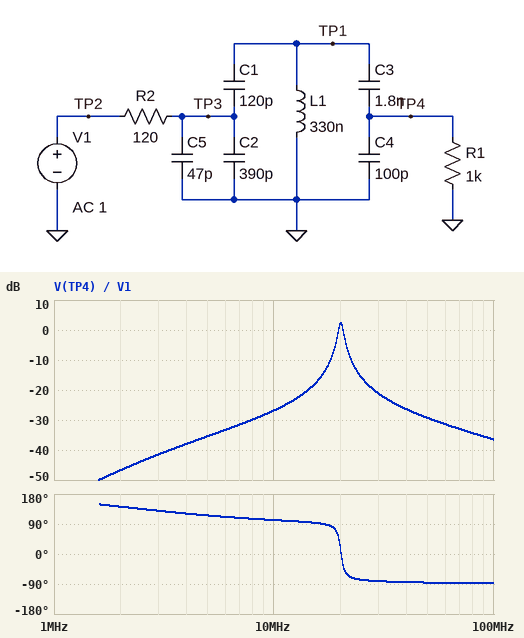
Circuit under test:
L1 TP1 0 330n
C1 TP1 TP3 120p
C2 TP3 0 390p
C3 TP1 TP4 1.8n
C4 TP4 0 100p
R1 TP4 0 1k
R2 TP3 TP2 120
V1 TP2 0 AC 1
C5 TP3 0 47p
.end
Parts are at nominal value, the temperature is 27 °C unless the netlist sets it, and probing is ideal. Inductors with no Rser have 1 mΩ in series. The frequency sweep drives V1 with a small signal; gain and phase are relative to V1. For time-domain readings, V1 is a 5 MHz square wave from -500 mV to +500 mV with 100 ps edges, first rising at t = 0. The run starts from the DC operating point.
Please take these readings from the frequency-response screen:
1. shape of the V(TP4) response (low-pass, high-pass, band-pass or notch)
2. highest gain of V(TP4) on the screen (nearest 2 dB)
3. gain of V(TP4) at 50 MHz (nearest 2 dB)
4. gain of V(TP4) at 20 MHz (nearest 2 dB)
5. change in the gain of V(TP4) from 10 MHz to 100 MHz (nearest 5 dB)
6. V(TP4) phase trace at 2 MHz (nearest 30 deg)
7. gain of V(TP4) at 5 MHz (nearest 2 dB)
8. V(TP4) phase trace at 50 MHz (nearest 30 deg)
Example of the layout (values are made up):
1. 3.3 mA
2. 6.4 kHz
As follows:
1. band-pass
2. 2 dB
3. -30 dB
4. 2 dB
5. -10 dB
6. 150 deg
7. -36 dB
8. -90 deg
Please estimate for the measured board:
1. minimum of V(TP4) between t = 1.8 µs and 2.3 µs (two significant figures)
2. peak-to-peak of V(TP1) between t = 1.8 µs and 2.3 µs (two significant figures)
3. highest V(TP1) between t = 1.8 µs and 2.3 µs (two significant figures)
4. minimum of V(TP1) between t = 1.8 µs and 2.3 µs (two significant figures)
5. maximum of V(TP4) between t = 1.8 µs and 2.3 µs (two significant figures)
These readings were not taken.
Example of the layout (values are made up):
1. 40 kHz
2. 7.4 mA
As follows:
1. -41 mV
2. 86 mV
3. 43 mV
4. -43 mV
5. 41 mV
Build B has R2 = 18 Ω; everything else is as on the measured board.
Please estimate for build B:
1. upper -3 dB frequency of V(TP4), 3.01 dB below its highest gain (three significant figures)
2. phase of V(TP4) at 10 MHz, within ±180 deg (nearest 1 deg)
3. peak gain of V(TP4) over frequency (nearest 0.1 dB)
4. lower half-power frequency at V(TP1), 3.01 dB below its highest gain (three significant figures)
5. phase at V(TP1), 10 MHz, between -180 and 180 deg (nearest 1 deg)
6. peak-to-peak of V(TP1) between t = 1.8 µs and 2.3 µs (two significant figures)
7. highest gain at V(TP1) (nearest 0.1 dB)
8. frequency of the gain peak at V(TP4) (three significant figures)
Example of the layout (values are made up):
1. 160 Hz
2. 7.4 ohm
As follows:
1. 20.7 MHz
2. 146 deg
3. 11.1 dB
4. 18.7 MHz
5. 145 deg
6. 450 mV
7. 11.6 dB
8. 19.6 MHz
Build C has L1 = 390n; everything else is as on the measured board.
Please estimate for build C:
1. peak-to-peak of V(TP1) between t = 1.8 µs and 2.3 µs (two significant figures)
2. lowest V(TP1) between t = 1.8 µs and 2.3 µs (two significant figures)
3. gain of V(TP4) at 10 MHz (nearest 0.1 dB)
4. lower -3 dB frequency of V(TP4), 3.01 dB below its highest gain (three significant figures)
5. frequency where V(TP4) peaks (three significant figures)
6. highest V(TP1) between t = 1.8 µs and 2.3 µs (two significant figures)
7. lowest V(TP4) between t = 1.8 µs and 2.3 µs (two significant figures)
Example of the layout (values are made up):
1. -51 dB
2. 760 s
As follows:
1. 100 mV
2. -52 mV
3. -24.8 dB
4. 18.0 MHz
5. 18.5 MHz
6. 52 mV
7. -49 mV
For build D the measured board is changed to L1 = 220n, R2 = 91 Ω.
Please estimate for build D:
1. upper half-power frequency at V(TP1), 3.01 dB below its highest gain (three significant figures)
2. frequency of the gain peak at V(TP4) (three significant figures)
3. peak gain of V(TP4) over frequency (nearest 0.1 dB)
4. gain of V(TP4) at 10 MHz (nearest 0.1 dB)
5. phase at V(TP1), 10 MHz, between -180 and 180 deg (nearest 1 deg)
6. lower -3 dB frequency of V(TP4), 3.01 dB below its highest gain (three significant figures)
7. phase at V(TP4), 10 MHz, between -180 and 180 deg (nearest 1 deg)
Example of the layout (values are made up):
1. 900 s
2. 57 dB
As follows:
1. 25.3 MHz
2. 24.7 MHz
3. 4.0 dB
4. -29.0 dB
5. 106 deg
6. 24.1 MHz
7. 107 deg
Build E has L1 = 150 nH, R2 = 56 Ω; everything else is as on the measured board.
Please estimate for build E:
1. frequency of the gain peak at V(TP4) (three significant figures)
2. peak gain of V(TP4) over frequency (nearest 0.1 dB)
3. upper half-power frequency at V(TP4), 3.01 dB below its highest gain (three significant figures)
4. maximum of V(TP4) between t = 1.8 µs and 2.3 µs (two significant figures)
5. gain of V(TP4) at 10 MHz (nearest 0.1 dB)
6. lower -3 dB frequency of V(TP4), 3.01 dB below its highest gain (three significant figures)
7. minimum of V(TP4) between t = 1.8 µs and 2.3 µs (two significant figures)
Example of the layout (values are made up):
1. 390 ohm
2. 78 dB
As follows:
1. 29.8 MHz
2. 6.5 dB
3. 30.6 MHz
4. 64 mV
5. -29.2 dB
6. 29.1 MHz
7. -64 mV
